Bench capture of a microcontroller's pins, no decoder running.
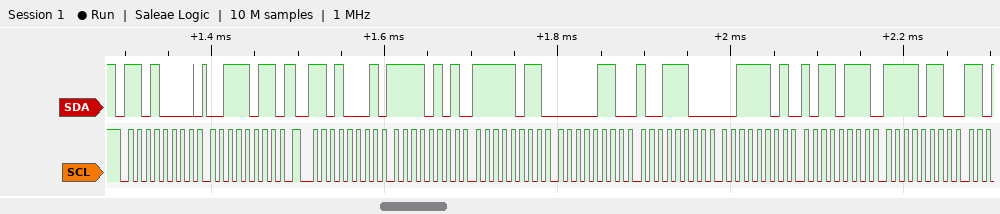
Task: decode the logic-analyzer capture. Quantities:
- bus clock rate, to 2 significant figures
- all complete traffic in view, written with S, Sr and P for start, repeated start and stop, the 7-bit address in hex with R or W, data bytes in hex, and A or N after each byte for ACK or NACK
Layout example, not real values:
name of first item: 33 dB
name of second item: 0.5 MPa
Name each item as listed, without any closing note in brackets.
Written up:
bus clock rate, to 2 significant figures: 100 kHz
all complete traffic in view, written with S, Sr and P for start, repeated start and stop, the 7-bit address in hex with R or W, data bytes in hex, and A or N after each byte for ACK or NACK: S 68W A 3B A Sr 68R A F5 A FB A 06 A 9C A 3D A B7 A F6 A
